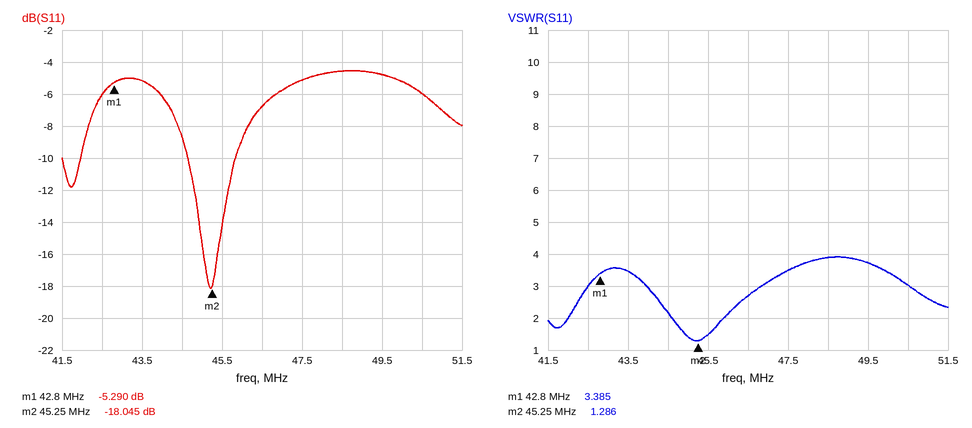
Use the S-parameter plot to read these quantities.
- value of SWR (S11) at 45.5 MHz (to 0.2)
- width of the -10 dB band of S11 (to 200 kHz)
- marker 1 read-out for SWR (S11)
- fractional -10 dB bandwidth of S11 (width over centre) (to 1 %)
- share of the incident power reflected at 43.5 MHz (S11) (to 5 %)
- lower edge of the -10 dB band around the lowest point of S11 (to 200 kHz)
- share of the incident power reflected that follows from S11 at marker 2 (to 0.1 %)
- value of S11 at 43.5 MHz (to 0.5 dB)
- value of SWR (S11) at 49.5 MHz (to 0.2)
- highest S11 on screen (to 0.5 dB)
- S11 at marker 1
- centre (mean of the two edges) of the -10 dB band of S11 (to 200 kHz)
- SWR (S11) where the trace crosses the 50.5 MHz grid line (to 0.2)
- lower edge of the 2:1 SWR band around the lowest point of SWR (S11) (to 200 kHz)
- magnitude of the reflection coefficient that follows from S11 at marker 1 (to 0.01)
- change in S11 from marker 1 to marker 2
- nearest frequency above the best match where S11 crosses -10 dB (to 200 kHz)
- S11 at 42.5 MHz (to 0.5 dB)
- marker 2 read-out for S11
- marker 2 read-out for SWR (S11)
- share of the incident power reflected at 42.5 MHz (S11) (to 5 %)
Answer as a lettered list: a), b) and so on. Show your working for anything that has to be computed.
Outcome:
a) 1.4
b) 45.8 MHz − 44.6 MHz = 1.2 MHz
c) 3.385
d) 1.2 MHz / 45.2 MHz ≈ 3 %
e) 10^(-5/10) ≈ 31.6 %, so 30 % to the nearest 5 %
f) 44.6 MHz
g) 10^(-18.045/10) ≈ 1.6 %
h) -5.0 dB
i) 3.8
j) -4.5 dB
k) -5.290 dB
l) 45.2 MHz
m) 3.0
n) 44.6 MHz
o) 10^(-5.29/20) ≈ 0.54
p) -18.045 − (-5.29) = -12.755 dB
q) 45.8 MHz
r) -6.0 dB
s) -18.045 dB
t) 1.286
u) 10^(-6/10) ≈ 25 %
